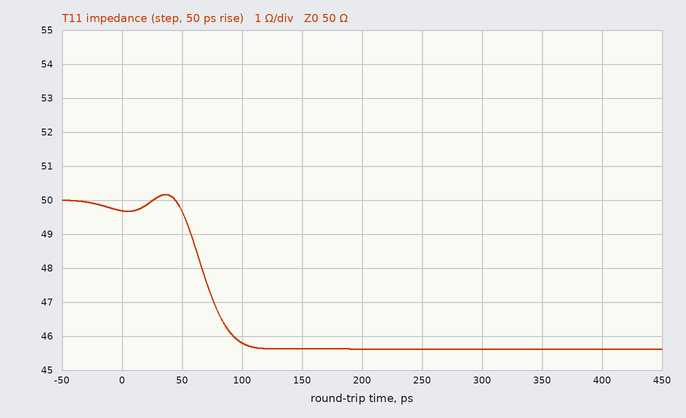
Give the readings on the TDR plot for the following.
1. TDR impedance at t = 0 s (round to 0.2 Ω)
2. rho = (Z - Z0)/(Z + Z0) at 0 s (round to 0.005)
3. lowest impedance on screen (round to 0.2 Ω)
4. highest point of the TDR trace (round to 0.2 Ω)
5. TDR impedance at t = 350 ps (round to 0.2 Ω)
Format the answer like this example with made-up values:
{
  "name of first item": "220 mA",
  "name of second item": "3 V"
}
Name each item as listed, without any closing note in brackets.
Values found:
{
  "TDR impedance at t = 0 s": "49.6 Ω",
  "rho = (Z - Z0)/(Z + Z0) at 0 s": "-0.005",
  "lowest impedance on screen": "45.6 Ω",
  "highest point of the TDR trace": "50.2 Ω",
  "TDR impedance at t = 350 ps": "45.6 Ω"
}
